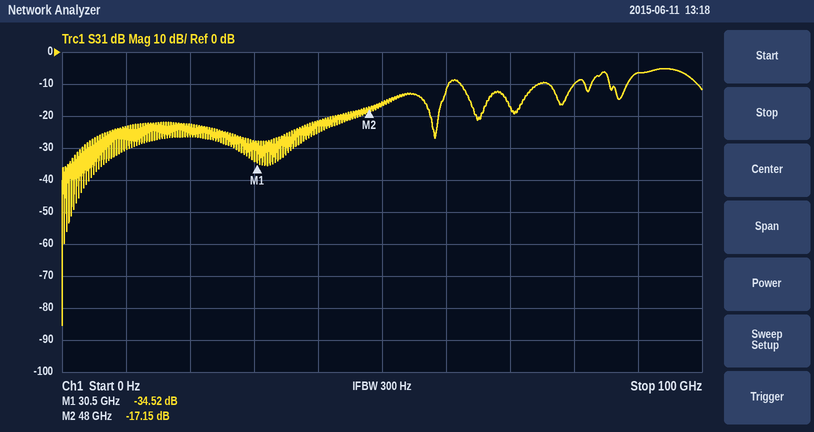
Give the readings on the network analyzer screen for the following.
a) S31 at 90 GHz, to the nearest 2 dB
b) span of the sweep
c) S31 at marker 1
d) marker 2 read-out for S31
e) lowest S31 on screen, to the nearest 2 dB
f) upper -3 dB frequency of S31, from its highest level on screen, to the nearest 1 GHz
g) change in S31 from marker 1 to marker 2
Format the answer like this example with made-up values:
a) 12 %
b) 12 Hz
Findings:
a) -6 dB
b) 100 GHz
c) -34.52 dB
d) -17.15 dB
e) -86 dB
f) 98 GHz
g) 17.37 dB
